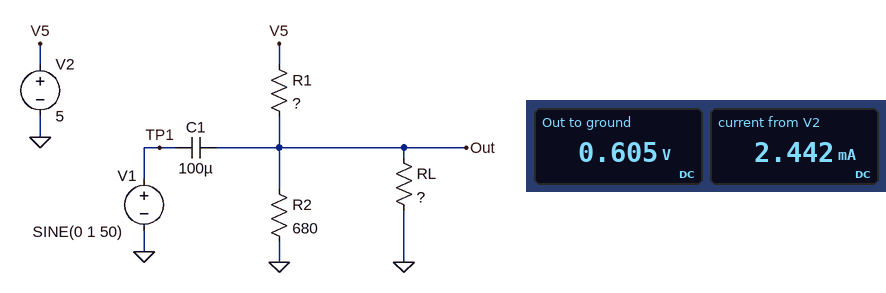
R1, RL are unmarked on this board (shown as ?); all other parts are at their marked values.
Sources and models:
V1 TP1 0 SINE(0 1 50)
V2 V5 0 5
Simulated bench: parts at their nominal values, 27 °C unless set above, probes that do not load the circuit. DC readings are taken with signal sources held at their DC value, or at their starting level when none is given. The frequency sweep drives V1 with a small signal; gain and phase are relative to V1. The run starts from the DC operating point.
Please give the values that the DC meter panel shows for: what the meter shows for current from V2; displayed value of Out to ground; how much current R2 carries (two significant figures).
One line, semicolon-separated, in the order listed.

2.442 mA; 0.605 V; 890 µA
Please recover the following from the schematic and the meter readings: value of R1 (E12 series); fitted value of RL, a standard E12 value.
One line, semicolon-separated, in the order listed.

1.8 kΩ; 390 Ω
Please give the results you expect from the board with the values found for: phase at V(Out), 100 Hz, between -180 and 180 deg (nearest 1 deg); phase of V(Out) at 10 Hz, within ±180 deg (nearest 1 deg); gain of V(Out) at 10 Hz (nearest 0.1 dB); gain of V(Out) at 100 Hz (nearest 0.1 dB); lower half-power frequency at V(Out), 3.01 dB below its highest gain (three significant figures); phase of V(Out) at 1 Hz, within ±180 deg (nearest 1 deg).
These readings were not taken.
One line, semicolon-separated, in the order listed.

4 deg; 36 deg; -1.9 dB; 0 dB; 7.31 Hz; 82 deg
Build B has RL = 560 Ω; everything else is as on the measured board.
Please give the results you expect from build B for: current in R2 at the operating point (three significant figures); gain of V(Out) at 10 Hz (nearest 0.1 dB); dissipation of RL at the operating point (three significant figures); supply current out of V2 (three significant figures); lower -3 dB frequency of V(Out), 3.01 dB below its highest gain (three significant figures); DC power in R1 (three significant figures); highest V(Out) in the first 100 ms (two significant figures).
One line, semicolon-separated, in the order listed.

1.07 mA; -1.4 dB; 948 µW; 2.37 mA; 6.07 Hz; 10.1 mW; 1.7 V
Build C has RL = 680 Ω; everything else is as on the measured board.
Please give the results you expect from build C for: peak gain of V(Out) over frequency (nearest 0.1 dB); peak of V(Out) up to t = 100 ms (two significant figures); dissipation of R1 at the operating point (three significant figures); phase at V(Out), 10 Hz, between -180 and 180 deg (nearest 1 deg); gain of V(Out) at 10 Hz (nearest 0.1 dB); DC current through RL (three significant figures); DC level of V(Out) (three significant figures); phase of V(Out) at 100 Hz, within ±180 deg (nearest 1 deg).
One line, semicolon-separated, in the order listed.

0 dB; 1.8 V; 9.83 mW; 29 deg; -1.2 dB; 1.17 mA; 794 mV; 3 deg
